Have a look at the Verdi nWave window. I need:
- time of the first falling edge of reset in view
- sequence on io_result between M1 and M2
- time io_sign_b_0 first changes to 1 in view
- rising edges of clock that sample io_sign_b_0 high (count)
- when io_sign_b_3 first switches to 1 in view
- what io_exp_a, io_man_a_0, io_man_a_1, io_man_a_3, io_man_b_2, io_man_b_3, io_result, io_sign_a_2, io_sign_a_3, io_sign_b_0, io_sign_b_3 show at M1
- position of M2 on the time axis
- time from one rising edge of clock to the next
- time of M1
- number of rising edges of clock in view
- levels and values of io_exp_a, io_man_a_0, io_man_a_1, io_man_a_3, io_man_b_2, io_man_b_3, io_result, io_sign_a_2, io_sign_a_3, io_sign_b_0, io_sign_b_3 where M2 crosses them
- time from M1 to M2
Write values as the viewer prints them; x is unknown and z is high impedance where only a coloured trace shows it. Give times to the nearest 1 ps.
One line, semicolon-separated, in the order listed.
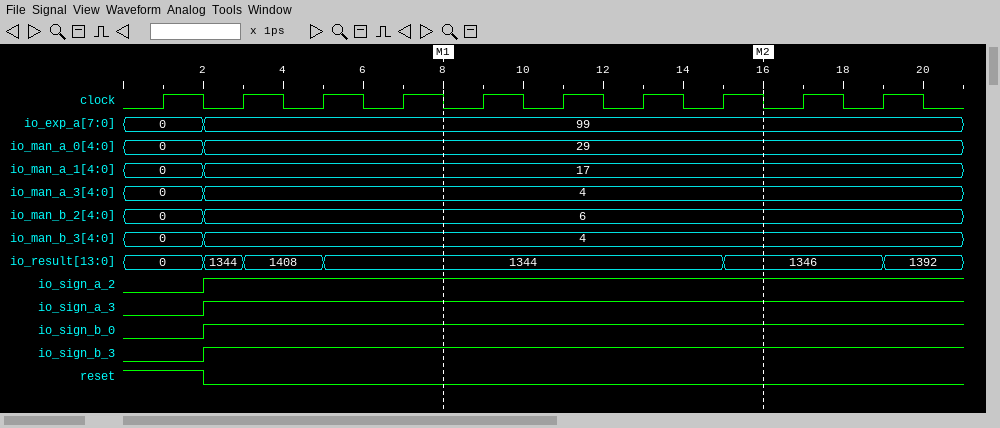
2 ps; 1344, 1346; 2 ps; 9; 2 ps; io_exp_a=99, io_man_a_0=29, io_man_a_1=17, io_man_a_3=4, io_man_b_2=6, io_man_b_3=4, io_result=1344, io_sign_a_2=1, io_sign_a_3=1, io_sign_b_0=1, io_sign_b_3=1; 16 ps; 2 ps; 8 ps; 10; io_exp_a=99, io_man_a_0=29, io_man_a_1=17, io_man_a_3=4, io_man_b_2=6, io_man_b_3=4, io_result=1346, io_sign_a_2=1, io_sign_a_3=1, io_sign_b_0=1, io_sign_b_3=1; 8 ps
